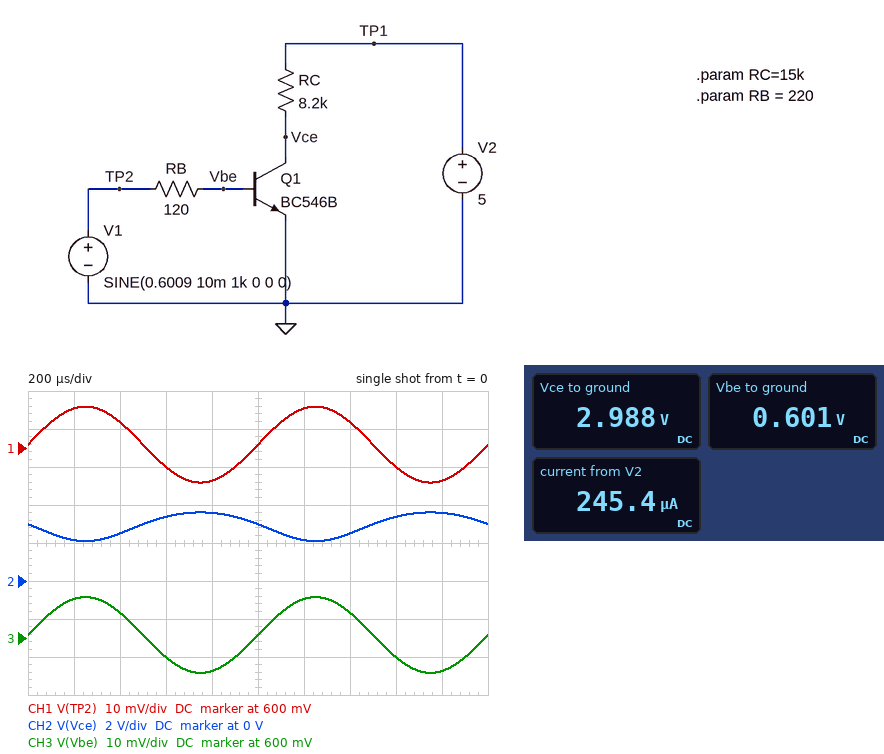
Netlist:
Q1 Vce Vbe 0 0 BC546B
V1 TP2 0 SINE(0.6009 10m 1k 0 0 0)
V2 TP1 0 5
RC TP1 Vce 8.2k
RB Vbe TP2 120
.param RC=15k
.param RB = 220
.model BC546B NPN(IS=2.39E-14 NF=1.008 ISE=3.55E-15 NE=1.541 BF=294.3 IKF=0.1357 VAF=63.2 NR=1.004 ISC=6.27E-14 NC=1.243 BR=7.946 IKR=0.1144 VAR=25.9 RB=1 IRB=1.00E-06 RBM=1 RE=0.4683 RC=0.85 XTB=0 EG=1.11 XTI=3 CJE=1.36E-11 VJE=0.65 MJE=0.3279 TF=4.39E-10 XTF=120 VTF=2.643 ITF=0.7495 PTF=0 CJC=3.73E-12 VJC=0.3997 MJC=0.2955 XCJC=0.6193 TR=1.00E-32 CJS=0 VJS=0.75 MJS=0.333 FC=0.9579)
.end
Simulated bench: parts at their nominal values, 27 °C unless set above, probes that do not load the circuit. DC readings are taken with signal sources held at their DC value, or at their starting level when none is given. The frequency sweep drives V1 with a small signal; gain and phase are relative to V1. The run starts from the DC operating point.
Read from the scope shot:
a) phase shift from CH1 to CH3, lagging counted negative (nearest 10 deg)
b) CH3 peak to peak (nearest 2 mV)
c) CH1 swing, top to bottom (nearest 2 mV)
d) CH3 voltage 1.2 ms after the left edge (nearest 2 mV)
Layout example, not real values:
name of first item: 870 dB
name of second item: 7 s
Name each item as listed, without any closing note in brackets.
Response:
phase shift from CH1 to CH3, lagging counted negative: 0 deg
CH3 peak to peak: 20 mV
CH1 swing, top to bottom: 20 mV
CH3 voltage 1.2 ms after the left edge: 610 mV
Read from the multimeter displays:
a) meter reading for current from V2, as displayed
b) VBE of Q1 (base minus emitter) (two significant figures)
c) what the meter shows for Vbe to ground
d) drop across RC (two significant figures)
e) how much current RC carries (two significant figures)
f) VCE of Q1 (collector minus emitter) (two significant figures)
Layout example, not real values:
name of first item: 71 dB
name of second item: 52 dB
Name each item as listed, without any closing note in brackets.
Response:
meter reading for current from V2, as displayed: 245.4 µA
VBE of Q1 (base minus emitter): 600 mV
what the meter shows for Vbe to ground: 0.601 V
drop across RC: 2.0 V
how much current RC carries: 250 µA
VCE of Q1 (collector minus emitter): 3.0 V
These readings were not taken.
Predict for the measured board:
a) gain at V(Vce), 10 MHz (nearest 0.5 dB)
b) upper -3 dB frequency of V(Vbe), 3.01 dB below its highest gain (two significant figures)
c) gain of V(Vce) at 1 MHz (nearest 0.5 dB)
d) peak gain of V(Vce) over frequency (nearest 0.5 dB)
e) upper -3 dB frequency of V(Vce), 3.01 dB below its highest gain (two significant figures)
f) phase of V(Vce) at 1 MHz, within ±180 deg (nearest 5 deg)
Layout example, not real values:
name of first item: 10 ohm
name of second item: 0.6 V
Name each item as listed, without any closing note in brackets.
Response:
gain at V(Vce), 10 MHz: 29.0 dB
upper -3 dB frequency of V(Vbe), 3.01 dB below its highest gain: 5.3 MHz
gain of V(Vce) at 1 MHz: 37.0 dB
peak gain of V(Vce) over frequency: 37.5 dB
upper -3 dB frequency of V(Vce), 3.01 dB below its highest gain: 4.2 MHz
phase of V(Vce) at 1 MHz, within ±180 deg: 165 deg
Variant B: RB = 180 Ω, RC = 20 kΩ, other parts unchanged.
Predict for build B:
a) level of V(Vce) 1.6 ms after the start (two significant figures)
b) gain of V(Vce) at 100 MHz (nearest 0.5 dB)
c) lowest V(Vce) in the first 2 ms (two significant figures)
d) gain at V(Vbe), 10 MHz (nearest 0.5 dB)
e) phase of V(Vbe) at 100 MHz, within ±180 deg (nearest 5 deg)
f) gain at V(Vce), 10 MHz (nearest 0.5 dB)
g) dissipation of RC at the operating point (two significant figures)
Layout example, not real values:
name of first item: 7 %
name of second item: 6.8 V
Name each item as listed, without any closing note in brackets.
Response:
level of V(Vce) 1.6 ms after the start: 1.2 V
gain of V(Vce) at 100 MHz: -5.0 dB
lowest V(Vce) in the first 2 ms: 46 mV
gain at V(Vbe), 10 MHz: -8.5 dB
phase of V(Vbe) at 100 MHz, within ±180 deg: -55 deg
gain at V(Vce), 10 MHz: 19.5 dB
dissipation of RC at the operating point: 1.1 mW
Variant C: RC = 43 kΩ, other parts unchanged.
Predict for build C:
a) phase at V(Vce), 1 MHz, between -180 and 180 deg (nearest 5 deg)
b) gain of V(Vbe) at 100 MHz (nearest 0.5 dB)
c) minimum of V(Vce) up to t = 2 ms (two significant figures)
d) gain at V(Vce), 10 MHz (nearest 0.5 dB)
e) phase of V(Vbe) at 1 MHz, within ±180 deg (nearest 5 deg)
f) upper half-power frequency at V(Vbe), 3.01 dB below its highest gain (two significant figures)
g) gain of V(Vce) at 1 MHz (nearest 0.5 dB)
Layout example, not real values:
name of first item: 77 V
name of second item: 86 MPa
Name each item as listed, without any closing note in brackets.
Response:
phase at V(Vce), 1 MHz, between -180 and 180 deg: 170 deg
gain of V(Vbe) at 100 MHz: -10.5 dB
minimum of V(Vce) up to t = 2 ms: 19 mV
gain at V(Vce), 10 MHz: -3.0 dB
phase of V(Vbe) at 1 MHz, within ±180 deg: -5 deg
upper half-power frequency at V(Vbe), 3.01 dB below its highest gain: 11 MHz
gain of V(Vce) at 1 MHz: -0.5 dB
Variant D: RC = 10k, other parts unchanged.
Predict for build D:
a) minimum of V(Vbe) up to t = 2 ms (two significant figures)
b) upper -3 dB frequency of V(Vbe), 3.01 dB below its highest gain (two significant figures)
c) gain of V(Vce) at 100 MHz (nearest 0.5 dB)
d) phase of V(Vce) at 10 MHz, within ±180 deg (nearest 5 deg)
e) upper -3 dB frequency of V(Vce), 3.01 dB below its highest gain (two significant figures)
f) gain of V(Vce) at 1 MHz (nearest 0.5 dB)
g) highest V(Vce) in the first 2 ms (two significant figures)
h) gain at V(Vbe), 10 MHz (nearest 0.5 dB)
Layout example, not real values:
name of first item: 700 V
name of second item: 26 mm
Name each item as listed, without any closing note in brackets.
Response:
minimum of V(Vbe) up to t = 2 ms: 590 mV
upper -3 dB frequency of V(Vbe), 3.01 dB below its highest gain: 4.3 MHz
gain of V(Vce) at 100 MHz: 5.5 dB
phase of V(Vce) at 10 MHz, within ±180 deg: 100 deg
upper -3 dB frequency of V(Vce), 3.01 dB below its highest gain: 3.3 MHz
gain of V(Vce) at 1 MHz: 38.5 dB
highest V(Vce) in the first 2 ms: 3.3 V
gain at V(Vbe), 10 MHz: -5.5 dB
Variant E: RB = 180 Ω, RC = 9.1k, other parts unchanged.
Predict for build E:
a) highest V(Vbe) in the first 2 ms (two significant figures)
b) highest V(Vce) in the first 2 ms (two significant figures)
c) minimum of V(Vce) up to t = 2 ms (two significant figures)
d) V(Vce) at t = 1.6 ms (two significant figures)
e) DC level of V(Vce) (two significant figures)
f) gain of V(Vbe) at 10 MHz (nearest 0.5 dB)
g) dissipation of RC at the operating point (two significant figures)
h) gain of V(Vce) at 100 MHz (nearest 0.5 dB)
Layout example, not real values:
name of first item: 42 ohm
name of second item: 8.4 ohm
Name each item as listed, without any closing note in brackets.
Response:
highest V(Vbe) in the first 2 ms: 610 mV
highest V(Vce) in the first 2 ms: 3.5 V
minimum of V(Vce) up to t = 2 ms: 1.8 V
V(Vce) at t = 1.6 ms: 3.2 V
DC level of V(Vce): 2.8 V
gain of V(Vbe) at 10 MHz: -7.5 dB
dissipation of RC at the operating point: 540 µW
gain of V(Vce) at 100 MHz: 3.0 dB
